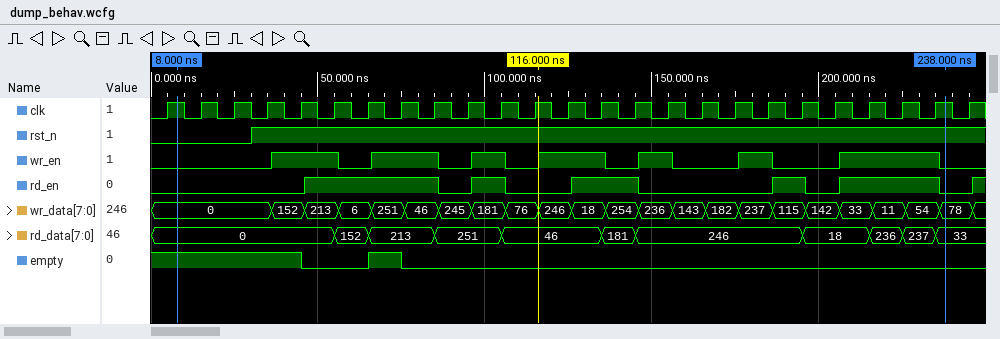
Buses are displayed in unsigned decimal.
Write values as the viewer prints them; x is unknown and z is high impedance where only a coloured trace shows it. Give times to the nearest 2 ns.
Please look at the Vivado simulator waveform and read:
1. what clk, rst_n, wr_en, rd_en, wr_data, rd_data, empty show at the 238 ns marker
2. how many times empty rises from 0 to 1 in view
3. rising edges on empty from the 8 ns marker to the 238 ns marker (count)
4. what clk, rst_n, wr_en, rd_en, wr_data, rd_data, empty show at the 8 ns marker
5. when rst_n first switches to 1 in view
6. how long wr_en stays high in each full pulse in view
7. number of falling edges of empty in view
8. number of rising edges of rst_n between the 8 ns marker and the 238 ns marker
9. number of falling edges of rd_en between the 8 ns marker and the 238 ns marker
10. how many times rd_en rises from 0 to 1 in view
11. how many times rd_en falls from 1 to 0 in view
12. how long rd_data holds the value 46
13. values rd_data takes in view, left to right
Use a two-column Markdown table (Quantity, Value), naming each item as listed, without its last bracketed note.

| Quantity | Value |
|---|---|
| what clk, rst_n, wr_en, rd_en, wr_data, rd_data, empty show at the 238 ns marker | clk=1, rst_n=1, wr_en=0, rd_en=0, wr_data=78, rd_data=33, empty=0 |
| how many times empty rises from 0 to 1 in view | 1 |
| rising edges on empty from the 8 ns marker to the 238 ns marker | 1 |
| what clk, rst_n, wr_en, rd_en, wr_data, rd_data, empty show at the 8 ns marker | clk=1, rst_n=0, wr_en=0, rd_en=0, wr_data=0, rd_data=0, empty=1 |
| when rst_n first switches to 1 in view | 30 ns |
| how long wr_en stays high in each full pulse in view | 20 ns, 20 ns, 10 ns, 20 ns, 10 ns, 10 ns, 30 ns |
| number of falling edges of empty in view | 2 |
| number of rising edges of rst_n between the 8 ns marker and the 238 ns marker | 1 |
| number of falling edges of rd_en between the 8 ns marker and the 238 ns marker | 5 |
| how many times rd_en rises from 0 to 1 in view | 6 |
| how many times rd_en falls from 1 to 0 in view | 5 |
| how long rd_data holds the value 46 | 30 ns |
| values rd_data takes in view, left to right | 0, 152, 213, 251, 46, 181, 246, 18, 236, 237, 33 |
